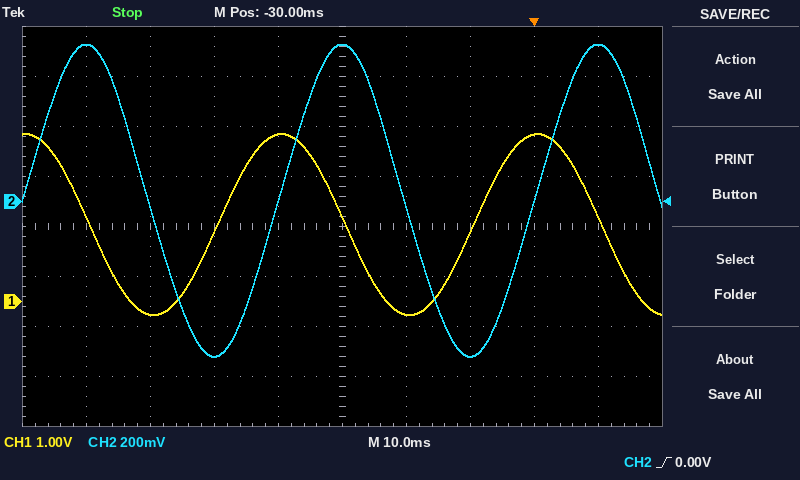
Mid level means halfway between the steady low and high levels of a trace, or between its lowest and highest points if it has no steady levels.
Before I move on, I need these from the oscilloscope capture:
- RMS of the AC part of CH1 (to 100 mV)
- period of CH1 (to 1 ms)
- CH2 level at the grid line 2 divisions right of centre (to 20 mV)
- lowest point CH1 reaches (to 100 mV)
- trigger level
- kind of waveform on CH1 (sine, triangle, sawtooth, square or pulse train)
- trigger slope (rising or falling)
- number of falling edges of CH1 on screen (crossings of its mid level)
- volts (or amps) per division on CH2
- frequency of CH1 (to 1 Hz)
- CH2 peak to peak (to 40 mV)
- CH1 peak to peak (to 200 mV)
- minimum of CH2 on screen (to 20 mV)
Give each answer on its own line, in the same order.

1.3 V
40 ms
-620 mV
-300 mV
0.00 V
sine
rising
3
200 mV
25 Hz
1.24 V
3.6 V
-620 mV
